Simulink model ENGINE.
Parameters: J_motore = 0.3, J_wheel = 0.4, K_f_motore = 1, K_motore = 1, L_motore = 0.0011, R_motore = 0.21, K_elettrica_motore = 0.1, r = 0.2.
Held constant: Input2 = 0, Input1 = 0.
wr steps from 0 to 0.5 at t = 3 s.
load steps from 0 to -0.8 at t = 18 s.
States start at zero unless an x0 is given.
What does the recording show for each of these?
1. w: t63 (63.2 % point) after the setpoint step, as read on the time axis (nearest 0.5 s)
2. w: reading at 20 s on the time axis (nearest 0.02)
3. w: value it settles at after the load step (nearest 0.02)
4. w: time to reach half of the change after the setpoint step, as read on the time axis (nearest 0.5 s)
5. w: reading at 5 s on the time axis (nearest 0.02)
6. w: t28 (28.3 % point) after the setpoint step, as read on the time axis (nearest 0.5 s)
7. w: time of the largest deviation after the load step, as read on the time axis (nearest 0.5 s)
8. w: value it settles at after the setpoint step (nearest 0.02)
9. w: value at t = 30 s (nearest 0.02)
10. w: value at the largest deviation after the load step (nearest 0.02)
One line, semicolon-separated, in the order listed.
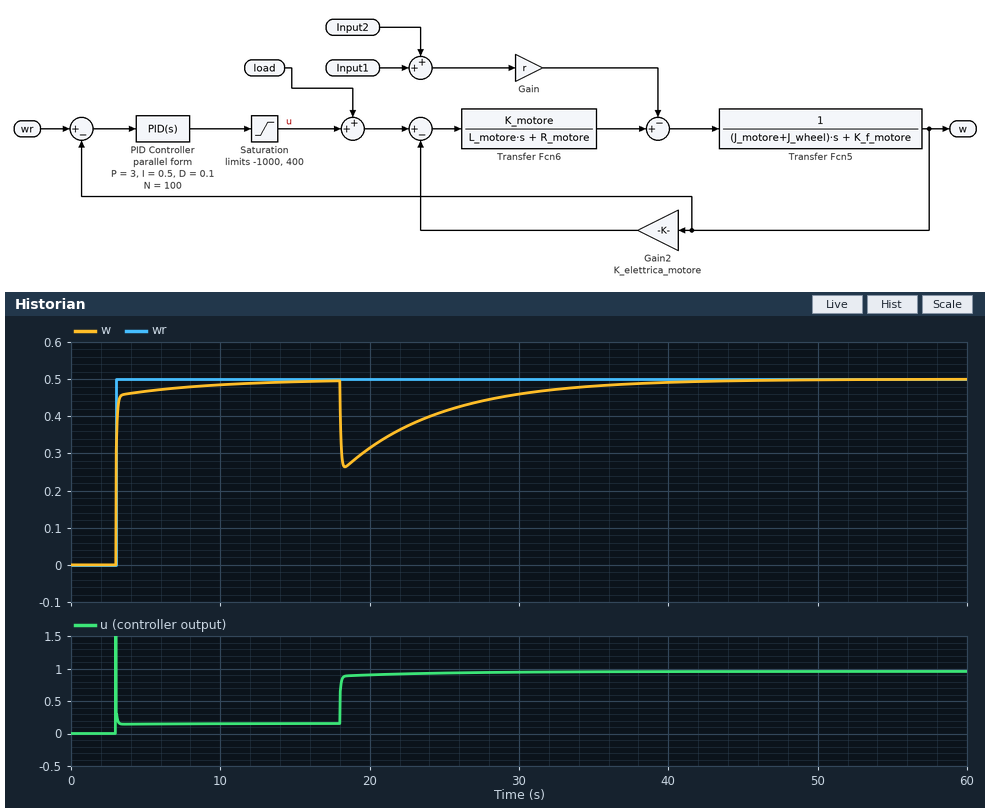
3.0 s; 0.32; 0.50; 3.0 s; 0.46; 3.0 s; 18.5 s; 0.50; 0.46; 0.26
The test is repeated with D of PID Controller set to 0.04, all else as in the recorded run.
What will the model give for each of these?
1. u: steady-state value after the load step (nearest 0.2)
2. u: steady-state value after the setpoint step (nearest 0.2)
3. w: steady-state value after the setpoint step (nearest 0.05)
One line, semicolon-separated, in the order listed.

1.0; 0.2; 0.50
